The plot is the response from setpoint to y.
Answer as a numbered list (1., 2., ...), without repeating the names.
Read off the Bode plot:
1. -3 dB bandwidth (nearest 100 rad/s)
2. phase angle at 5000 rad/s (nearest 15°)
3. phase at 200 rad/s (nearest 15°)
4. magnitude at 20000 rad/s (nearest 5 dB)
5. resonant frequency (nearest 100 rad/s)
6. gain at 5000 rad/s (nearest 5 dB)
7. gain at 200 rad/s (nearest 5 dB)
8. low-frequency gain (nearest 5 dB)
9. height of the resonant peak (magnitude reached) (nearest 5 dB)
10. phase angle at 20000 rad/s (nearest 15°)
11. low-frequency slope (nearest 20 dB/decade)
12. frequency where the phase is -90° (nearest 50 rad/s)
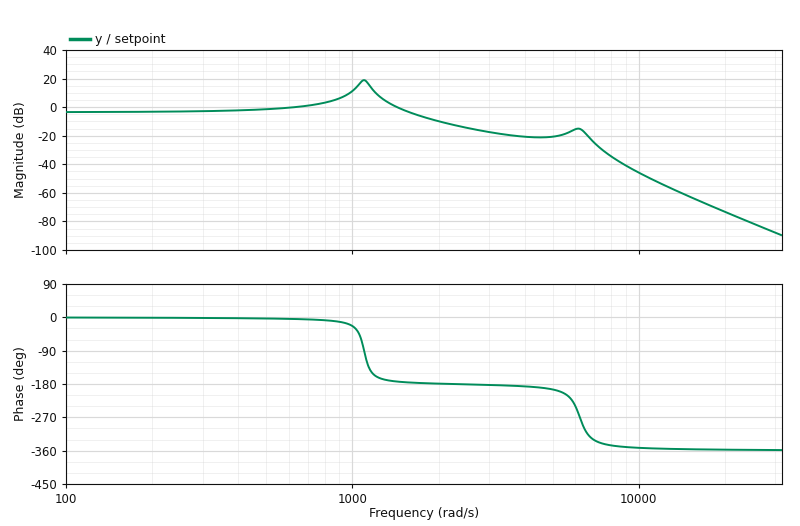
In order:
1. 1700 rad/s
2. -195°
3. 0°
4. -75 dB
5. 1100 rad/s
6. -20 dB
7. -5 dB
8. -5 dB
9. 20 dB
10. -360°
11. 0 dB/decade
12. 1100 rad/s
